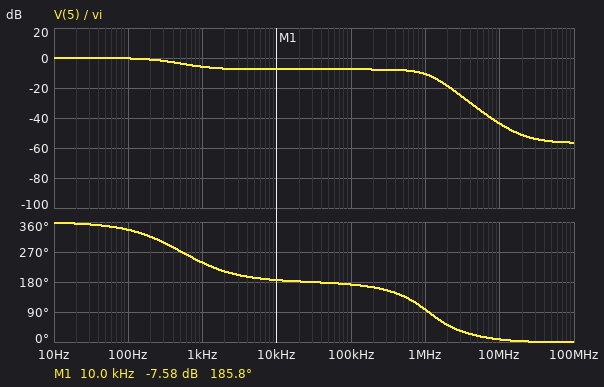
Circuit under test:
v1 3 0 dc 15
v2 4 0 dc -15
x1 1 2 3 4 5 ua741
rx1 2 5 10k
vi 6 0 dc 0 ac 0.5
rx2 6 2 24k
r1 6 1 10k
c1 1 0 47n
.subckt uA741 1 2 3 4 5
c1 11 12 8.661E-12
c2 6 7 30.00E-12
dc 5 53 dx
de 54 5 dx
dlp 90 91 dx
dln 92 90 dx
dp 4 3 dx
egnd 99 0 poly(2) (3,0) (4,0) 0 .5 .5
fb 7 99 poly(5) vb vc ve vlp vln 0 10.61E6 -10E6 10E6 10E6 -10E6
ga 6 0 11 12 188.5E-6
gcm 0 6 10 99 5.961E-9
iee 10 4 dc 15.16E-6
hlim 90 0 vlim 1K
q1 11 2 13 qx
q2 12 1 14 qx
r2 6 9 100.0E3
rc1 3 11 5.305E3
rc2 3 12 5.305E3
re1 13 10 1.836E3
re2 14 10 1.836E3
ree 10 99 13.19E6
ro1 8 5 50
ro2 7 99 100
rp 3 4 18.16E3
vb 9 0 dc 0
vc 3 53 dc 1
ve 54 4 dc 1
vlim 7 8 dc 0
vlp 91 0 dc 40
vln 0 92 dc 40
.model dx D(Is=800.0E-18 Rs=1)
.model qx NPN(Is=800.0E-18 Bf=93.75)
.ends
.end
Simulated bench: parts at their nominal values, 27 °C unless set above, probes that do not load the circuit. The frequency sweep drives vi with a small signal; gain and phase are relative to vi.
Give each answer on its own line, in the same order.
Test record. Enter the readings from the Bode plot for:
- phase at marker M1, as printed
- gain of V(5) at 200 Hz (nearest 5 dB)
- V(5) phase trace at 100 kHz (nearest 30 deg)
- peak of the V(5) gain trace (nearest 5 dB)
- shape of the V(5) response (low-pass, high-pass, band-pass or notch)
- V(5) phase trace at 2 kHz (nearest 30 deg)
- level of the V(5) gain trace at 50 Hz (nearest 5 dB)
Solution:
185.8 deg
0 dB
180 deg
0 dB
low-pass
210 deg
0 dB
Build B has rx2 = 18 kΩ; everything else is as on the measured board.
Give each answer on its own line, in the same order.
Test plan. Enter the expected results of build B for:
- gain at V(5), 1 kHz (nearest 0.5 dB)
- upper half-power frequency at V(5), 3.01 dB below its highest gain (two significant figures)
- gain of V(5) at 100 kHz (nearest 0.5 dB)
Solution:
-4.0 dB
550 Hz
-5.0 dB
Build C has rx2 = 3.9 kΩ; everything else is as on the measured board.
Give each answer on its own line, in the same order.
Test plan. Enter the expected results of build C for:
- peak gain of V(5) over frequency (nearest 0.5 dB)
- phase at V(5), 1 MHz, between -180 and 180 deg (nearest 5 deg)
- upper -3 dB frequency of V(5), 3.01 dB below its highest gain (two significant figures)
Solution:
8.0 dB
75 deg
330 kHz
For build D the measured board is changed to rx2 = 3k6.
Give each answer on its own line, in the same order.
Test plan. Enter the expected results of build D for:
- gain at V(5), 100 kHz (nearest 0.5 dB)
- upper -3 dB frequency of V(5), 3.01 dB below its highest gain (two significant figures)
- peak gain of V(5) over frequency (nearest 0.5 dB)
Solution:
8.5 dB
310 kHz
9.0 dB
